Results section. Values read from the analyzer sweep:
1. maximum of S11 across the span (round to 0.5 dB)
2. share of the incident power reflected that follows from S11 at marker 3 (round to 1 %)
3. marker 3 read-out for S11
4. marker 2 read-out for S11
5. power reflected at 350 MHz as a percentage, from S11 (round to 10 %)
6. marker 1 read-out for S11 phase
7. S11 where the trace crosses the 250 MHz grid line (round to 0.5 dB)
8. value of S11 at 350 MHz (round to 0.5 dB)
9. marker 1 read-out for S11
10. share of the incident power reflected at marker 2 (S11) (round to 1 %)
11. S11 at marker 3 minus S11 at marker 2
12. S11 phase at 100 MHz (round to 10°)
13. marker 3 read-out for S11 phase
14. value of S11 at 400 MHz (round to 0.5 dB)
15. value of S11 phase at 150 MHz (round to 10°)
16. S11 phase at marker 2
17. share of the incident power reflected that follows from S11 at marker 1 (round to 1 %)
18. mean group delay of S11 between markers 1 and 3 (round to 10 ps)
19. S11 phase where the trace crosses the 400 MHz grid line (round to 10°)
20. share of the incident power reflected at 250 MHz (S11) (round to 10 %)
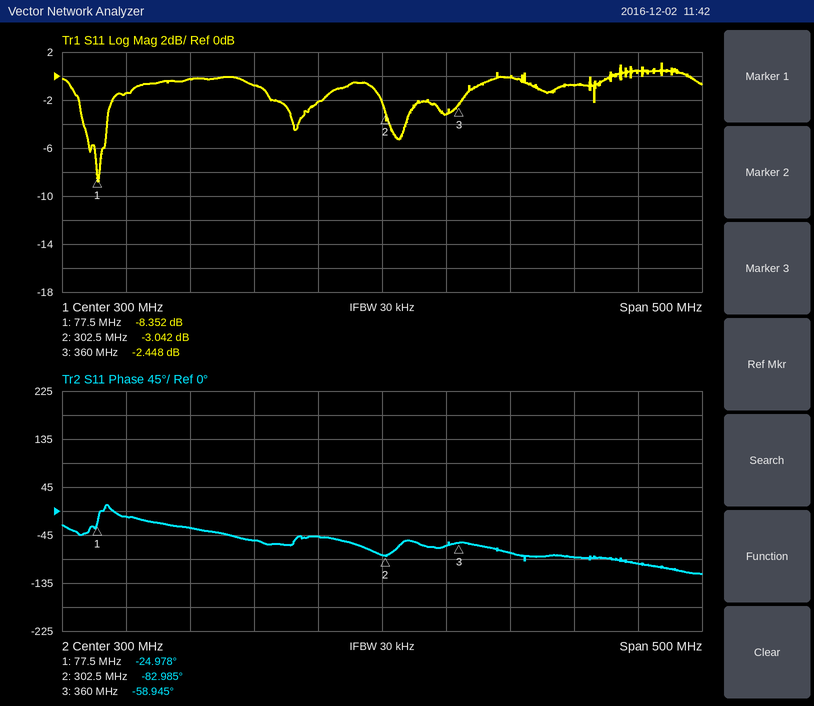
1.0 dB
57 %
-2.448 dB
-3.042 dB
50 %
-24.978°
-2.0 dB
-3.0 dB
-8.352 dB
50 %
0.594 dB
-10°
-58.945°
0.0 dB
-30°
-82.985°
15 %
330 ps
-80°
60 %
